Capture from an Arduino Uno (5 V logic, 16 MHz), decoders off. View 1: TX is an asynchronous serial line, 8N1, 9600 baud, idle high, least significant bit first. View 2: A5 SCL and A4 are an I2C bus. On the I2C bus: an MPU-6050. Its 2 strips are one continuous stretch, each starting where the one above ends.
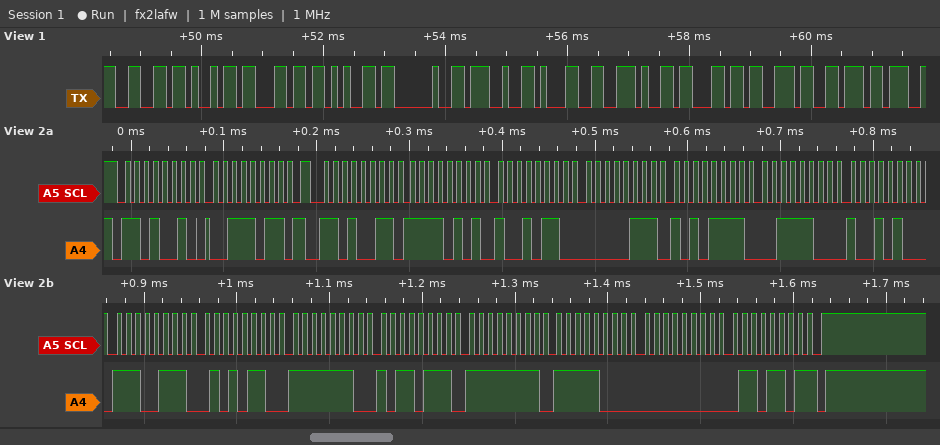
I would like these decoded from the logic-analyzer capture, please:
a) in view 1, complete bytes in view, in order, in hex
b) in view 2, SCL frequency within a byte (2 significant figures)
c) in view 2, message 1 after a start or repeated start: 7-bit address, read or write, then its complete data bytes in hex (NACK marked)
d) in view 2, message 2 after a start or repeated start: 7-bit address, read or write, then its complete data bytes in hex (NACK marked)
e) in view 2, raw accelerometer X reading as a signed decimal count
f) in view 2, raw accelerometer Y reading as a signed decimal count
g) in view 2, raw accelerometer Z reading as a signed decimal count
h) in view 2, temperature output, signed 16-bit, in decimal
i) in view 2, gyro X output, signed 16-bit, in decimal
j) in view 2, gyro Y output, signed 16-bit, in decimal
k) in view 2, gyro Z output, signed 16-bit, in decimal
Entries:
66 69 6C 65 20 27 31 2E 63 73 76
100 kHz
0x69 write: 3B
0x69 read: F5 96 07 AF 3C 94 E7 56 FE B7 FF F8 00 6D NACK
-2666
1967
15508
-6314
-329
-8
109
